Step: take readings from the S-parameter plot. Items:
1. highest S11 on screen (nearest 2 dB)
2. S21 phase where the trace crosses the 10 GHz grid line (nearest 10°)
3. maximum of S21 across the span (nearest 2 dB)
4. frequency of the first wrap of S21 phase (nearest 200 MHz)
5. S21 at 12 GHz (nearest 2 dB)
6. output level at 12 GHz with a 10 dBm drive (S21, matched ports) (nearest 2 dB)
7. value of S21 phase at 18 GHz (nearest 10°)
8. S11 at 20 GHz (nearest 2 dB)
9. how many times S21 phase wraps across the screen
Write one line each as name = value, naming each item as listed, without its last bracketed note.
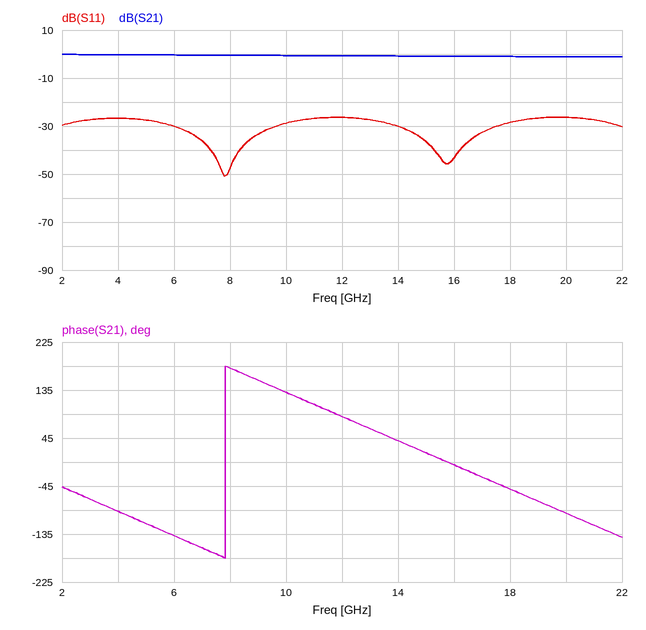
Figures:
highest S11 on screen = -26 dB
S21 phase where the trace crosses the 10 GHz grid line = 130°
maximum of S21 across the span = 0 dB
frequency of the first wrap of S21 phase = 7.8 GHz
S21 at 12 GHz = 0 dB
output level at 12 GHz with a 10 dBm drive (S21, matched ports) = 10 dBm
value of S21 phase at 18 GHz = -50°
S11 at 20 GHz = -26 dB
how many times S21 phase wraps across the screen = 1
